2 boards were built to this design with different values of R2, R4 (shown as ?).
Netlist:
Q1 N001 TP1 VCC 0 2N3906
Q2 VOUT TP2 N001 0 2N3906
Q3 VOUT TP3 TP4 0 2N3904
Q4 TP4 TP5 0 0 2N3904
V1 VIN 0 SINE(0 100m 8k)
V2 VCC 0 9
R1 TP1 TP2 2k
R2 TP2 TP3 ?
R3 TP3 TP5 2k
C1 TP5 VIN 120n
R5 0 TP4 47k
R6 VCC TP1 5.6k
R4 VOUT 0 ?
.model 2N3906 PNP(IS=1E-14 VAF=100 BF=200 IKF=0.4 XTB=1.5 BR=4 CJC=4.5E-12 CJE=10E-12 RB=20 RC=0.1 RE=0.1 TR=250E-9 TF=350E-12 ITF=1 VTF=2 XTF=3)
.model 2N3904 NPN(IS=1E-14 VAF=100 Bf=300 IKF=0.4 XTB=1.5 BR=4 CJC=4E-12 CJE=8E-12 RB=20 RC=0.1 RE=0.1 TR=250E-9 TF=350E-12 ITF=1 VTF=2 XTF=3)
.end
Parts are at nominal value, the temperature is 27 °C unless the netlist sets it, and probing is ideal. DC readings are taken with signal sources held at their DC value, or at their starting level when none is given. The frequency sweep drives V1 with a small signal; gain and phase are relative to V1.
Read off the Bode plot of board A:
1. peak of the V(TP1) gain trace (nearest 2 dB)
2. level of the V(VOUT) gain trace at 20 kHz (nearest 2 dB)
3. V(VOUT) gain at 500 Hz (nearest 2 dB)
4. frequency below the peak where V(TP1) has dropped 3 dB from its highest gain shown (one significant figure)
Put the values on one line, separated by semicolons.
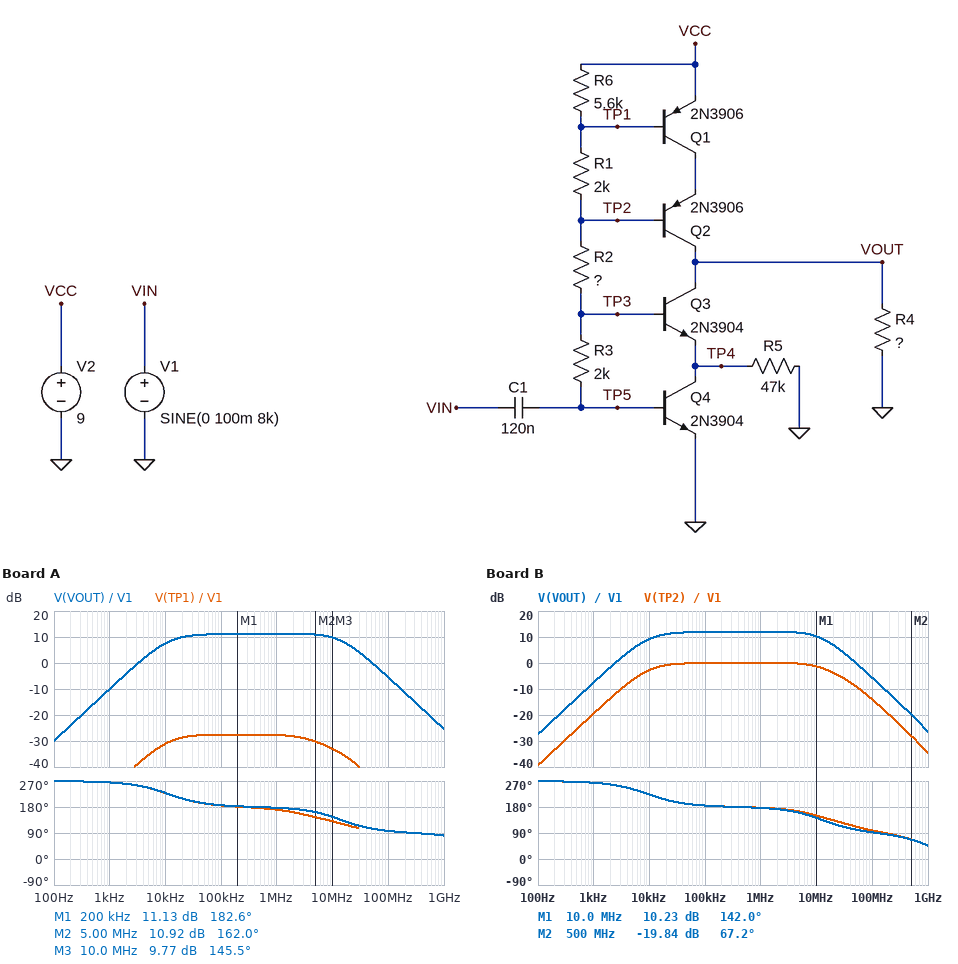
-28 dB; 10 dB; -16 dB; 10 kHz
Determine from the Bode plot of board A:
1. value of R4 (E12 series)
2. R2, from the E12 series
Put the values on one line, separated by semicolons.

2.7 Ω; 1 kΩ
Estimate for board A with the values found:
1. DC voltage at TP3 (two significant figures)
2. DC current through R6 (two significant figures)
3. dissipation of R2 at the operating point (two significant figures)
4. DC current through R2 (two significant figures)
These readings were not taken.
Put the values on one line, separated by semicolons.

1.2 V; 150 µA; 11 mW; 3.4 mA
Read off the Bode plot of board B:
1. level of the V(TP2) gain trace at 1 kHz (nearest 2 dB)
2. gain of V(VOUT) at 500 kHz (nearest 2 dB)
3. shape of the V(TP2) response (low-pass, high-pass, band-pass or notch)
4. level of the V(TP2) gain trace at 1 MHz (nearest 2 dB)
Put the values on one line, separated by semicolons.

-20 dB; 12 dB; band-pass; 0 dB
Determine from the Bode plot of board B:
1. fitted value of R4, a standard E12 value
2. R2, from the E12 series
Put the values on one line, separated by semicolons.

3.9 Ω; 3.3 kΩ
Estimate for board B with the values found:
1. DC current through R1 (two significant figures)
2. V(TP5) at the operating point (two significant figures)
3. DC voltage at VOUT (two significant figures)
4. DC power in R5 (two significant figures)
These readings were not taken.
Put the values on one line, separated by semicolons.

910 µA; 760 mV; 320 mV; 1.4 µW
